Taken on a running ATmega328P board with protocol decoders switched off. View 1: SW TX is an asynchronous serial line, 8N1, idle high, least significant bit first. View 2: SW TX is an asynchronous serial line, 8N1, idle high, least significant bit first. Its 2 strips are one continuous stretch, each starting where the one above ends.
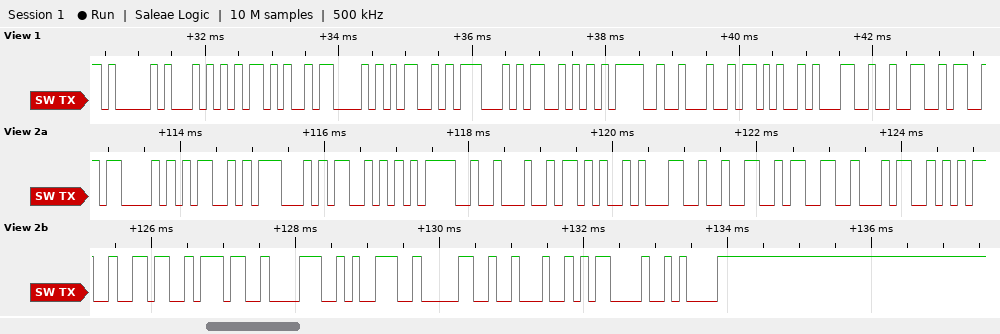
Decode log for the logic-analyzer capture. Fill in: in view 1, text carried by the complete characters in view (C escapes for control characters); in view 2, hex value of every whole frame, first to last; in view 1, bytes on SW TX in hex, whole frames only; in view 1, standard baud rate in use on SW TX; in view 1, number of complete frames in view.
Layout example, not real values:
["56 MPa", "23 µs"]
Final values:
["\"AT+CMGS=\\\"+12\"", "43 4D 47 53 3D 22 2B 31 32 33 34 35 36 37 38 39 30 22 0D 0A", "41 54 2B 43 4D 47 53 3D 22 2B 31 32", "9600 baud", "12"]
